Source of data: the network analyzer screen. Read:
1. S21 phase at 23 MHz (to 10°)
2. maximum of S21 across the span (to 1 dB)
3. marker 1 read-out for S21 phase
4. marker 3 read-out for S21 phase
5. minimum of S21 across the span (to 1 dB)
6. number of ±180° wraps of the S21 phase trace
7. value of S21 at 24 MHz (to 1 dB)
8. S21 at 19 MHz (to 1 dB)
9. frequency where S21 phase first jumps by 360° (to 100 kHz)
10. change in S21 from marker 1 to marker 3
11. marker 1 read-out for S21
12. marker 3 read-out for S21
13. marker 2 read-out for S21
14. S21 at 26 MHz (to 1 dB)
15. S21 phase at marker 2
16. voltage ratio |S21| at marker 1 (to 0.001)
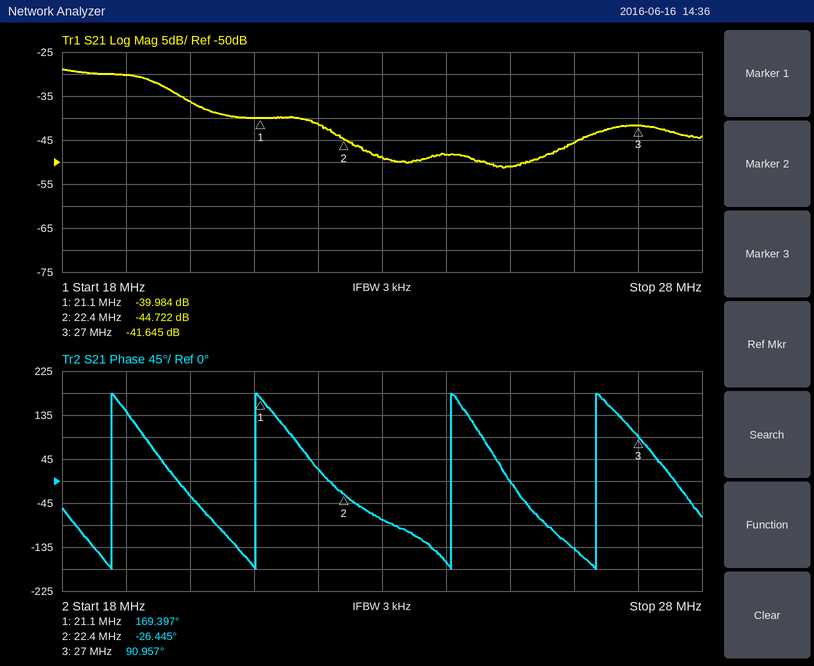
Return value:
-80°
-29 dB
169.397°
90.957°
-51 dB
4
-48 dB
-30 dB
18.8 MHz
-1.661 dB
-39.984 dB
-41.645 dB
-44.722 dB
-46 dB
-26.445°
0.010
